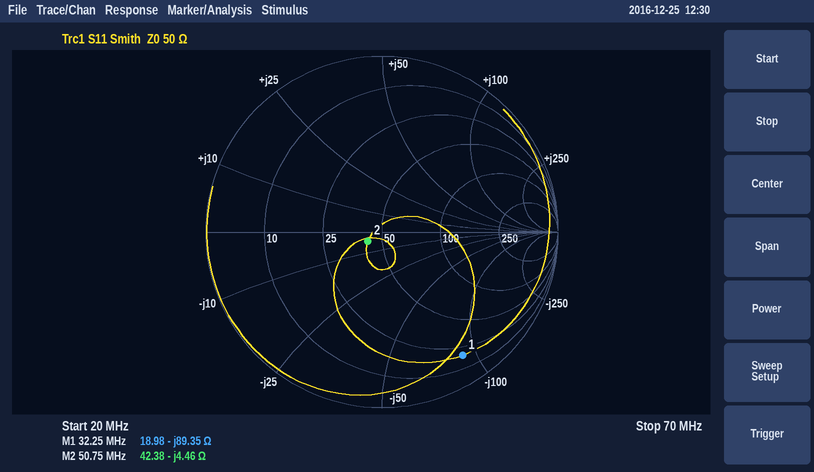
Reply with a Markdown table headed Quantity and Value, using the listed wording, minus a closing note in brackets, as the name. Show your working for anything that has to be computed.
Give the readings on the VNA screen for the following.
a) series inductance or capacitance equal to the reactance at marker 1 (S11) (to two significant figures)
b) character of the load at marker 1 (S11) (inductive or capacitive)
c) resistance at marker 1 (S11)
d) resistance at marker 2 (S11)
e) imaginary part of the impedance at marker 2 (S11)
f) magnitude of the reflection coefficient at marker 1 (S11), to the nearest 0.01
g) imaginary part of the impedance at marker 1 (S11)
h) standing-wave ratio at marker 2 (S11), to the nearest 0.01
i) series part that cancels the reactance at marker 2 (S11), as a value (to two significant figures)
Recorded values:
| Quantity | Value |
|---|---|
| series inductance or capacitance equal to the reactance at marker 1 (S11) | C = 1/(2π × 32.25 MHz × 89.35 Ω) ≈ 55 pF |
| character of the load at marker 1 (S11) | capacitive |
| resistance at marker 1 | 18.98 Ω |
| resistance at marker 2 | 42.38 Ω |
| imaginary part of the impedance at marker 2 | -4.46 Ω |
| magnitude of the reflection coefficient at marker 1 (S11), to the nearest 0.01 | 0.84 |
| imaginary part of the impedance at marker 1 | -89.35 Ω |
| standing-wave ratio at marker 2 (S11), to the nearest 0.01 | 1.21 |
| series part that cancels the reactance at marker 2 (S11), as a value | L = 4.46 Ω/(2π × 50.75 MHz) ≈ 14 nH |
